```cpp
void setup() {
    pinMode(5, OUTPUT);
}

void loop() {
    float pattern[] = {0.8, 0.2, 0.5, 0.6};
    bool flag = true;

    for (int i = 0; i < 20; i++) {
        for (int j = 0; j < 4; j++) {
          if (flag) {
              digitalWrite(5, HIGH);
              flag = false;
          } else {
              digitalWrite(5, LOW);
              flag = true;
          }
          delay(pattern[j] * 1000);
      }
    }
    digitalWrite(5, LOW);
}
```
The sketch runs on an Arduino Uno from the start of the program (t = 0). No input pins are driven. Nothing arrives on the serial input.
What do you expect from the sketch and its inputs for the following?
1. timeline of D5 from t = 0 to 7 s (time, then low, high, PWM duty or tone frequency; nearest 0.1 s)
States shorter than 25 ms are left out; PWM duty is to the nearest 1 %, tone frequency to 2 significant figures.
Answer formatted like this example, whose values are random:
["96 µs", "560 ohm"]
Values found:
["0 s high; 0.8 s low; 1 s high; 1.5 s low; 2.1 s high; 2.9 s low; 3.1 s high; 3.6 s low; 4.2 s high; 5 s low; 5.2 s high; 5.7 s low; 6.3 s high"]
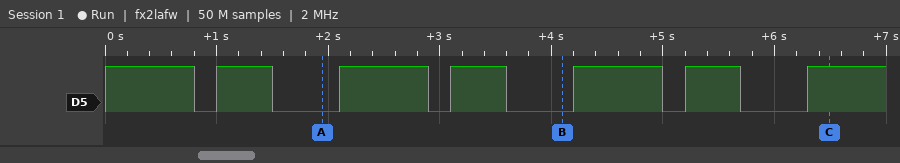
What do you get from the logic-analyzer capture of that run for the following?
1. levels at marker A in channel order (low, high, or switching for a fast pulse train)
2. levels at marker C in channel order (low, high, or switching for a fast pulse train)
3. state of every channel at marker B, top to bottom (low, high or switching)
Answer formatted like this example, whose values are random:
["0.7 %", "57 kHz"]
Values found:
["D5 low", "D5 high", "D5 low"]
